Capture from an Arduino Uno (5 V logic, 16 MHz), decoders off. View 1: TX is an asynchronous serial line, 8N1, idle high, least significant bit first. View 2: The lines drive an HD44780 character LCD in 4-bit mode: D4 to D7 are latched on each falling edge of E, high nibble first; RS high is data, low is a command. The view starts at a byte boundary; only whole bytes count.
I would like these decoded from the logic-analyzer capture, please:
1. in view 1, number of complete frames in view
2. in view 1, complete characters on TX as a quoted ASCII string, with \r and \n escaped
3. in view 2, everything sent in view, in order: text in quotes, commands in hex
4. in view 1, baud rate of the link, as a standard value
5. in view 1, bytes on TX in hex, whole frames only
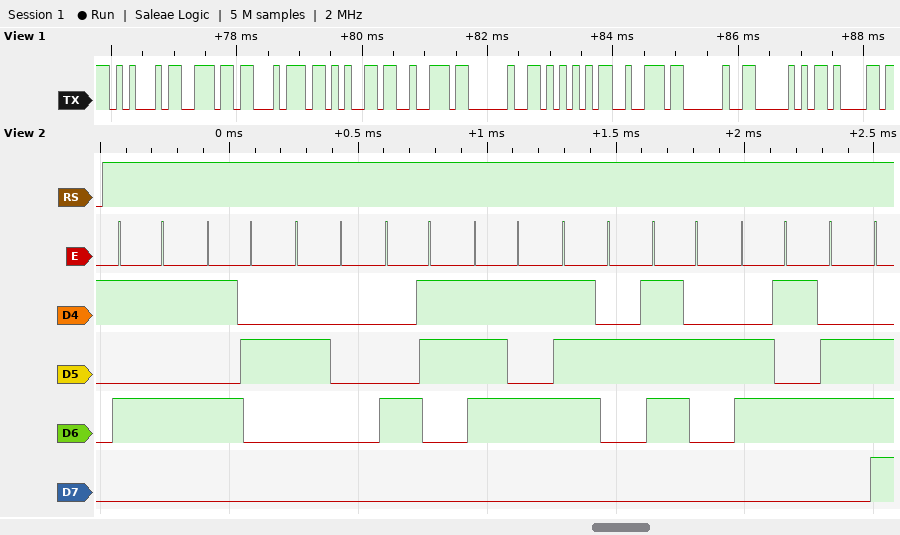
11
"Enter Ur Pa"
"UR Curren"
9600 baud
45 6E 74 65 72 20 55 72 20 50 61
